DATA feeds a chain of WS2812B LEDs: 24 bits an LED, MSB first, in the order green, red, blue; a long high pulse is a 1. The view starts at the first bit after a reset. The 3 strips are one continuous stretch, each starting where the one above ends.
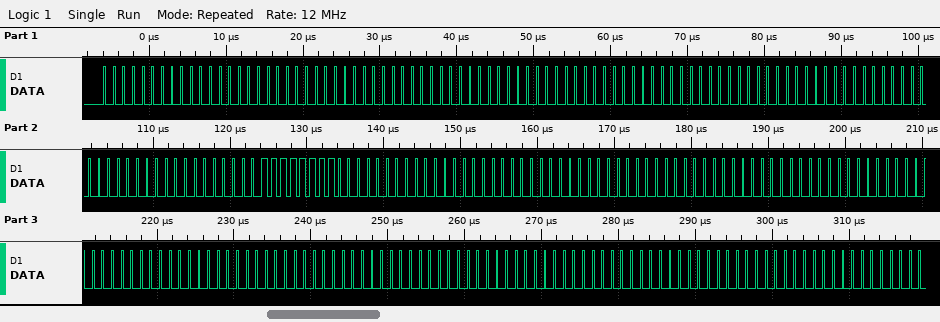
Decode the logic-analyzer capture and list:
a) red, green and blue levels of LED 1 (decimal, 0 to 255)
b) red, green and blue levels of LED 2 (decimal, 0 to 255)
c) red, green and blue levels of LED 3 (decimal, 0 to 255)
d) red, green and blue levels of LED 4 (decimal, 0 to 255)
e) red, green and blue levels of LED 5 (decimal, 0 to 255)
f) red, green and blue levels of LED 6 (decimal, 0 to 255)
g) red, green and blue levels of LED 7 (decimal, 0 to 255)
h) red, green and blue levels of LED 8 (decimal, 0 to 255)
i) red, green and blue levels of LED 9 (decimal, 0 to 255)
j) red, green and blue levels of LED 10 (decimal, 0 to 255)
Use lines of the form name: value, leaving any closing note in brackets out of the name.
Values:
red, green and blue levels of LED 1: 0, 0, 0
red, green and blue levels of LED 2: 0, 0, 0
red, green and blue levels of LED 3: 0, 0, 0
red, green and blue levels of LED 4: 0, 0, 0
red, green and blue levels of LED 5: 255, 0, 0
red, green and blue levels of LED 6: 0, 0, 0
red, green and blue levels of LED 7: 0, 0, 0
red, green and blue levels of LED 8: 0, 0, 0
red, green and blue levels of LED 9: 0, 0, 0
red, green and blue levels of LED 10: 0, 0, 0
